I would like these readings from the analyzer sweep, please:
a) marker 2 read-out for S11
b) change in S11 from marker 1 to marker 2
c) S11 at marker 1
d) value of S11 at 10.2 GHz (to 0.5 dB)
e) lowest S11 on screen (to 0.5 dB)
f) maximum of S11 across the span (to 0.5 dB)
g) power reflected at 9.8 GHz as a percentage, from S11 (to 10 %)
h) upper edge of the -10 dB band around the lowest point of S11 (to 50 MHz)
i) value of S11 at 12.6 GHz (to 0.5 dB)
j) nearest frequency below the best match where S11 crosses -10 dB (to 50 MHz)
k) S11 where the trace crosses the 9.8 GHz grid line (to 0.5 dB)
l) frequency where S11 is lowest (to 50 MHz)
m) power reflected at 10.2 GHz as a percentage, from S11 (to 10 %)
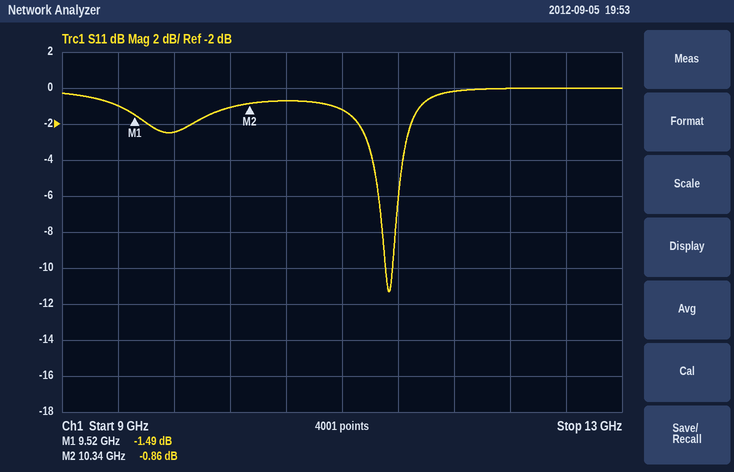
-0.86 dB
0.63 dB
-1.49 dB
-1.0 dB
-11.5 dB
0.0 dB
60 %
11.35 GHz
0.0 dB
11.30 GHz
-2.5 dB
11.35 GHz
80 %
